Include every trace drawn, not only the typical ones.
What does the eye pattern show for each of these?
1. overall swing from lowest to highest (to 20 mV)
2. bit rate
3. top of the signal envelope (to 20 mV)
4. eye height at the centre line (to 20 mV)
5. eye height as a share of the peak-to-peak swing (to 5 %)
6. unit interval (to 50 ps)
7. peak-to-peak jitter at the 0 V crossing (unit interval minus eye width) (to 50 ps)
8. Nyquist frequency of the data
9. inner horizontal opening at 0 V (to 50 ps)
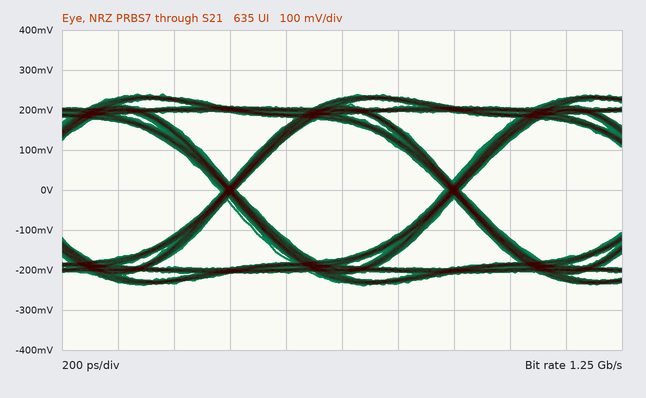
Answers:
480 mV
1.25 Gb/s
240 mV
340 mV
70 %
800 ps
50 ps
625 MHz
750 ps
